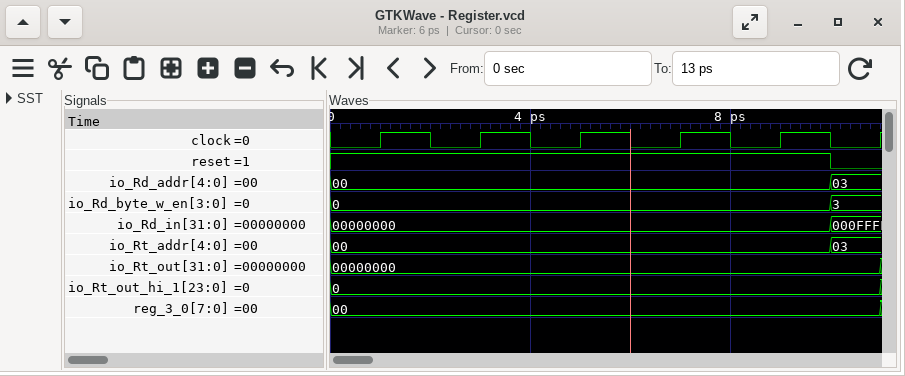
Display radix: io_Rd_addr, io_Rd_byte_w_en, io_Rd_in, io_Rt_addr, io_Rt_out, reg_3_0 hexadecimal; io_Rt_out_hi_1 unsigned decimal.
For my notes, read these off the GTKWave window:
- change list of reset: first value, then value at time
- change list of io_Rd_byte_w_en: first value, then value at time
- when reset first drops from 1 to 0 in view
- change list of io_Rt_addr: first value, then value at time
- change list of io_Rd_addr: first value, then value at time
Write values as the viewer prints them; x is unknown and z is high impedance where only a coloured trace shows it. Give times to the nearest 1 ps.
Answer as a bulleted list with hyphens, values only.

- 1, 0 at 10 ps
- 0, 3 at 10 ps
- 10 ps
- 00, 03 at 10 ps
- 00, 03 at 10 ps
